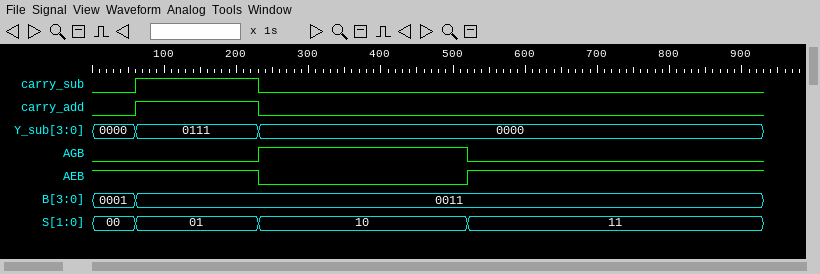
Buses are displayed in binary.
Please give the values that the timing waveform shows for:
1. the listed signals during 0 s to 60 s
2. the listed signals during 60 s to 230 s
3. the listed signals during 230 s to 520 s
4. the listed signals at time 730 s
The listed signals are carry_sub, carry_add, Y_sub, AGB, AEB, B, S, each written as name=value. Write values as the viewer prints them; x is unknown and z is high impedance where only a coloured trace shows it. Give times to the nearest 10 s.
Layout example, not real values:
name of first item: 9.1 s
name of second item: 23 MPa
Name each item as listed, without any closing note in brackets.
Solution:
the listed signals during 0 s to 60 s: carry_sub=0, carry_add=0, Y_sub=0000, AGB=0, AEB=1, B=0001, S=00
the listed signals during 60 s to 230 s: carry_sub=1, carry_add=1, Y_sub=0111, AGB=0, AEB=1, B=0011, S=01
the listed signals during 230 s to 520 s: carry_sub=0, carry_add=0, Y_sub=0000, AGB=1, AEB=0, B=0011, S=10
the listed signals at time 730 s: carry_sub=0, carry_add=0, Y_sub=0000, AGB=0, AEB=1, B=0011, S=11
